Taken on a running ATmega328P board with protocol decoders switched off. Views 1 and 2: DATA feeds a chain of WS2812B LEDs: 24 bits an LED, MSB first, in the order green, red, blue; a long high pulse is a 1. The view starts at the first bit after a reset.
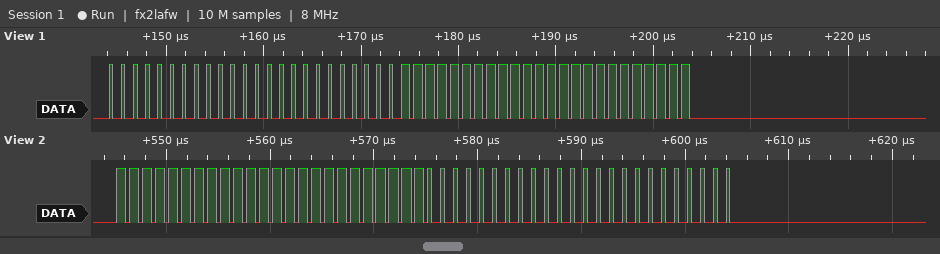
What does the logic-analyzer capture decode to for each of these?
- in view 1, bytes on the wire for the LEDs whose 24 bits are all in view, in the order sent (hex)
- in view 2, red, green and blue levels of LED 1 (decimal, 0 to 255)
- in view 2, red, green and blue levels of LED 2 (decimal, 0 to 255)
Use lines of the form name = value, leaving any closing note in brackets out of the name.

in view 1, bytes on the wire for the LEDs whose 24 bits are all in view, in the order sent = 00 00 00 FF FF FF
in view 2, red, green and blue levels of LED 1 = 255, 255, 255
in view 2, red, green and blue levels of LED 2 = 0, 0, 0
